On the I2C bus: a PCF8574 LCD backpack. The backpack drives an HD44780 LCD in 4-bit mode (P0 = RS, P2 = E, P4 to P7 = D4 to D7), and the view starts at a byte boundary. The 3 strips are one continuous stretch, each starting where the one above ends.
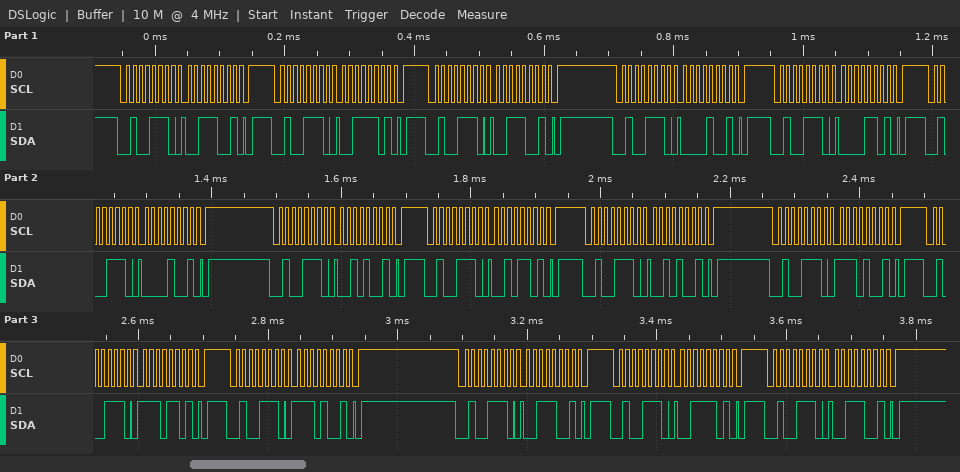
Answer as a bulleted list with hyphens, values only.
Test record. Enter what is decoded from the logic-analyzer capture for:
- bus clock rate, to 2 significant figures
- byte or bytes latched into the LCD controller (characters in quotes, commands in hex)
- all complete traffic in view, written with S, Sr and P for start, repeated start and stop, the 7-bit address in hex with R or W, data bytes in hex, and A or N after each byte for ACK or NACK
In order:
- 100 kHz
- '0' '.'
- S 27W A 39 A P S 27W A 3D A P S 27W A 39 A P S 27W A 09 A P S 27W A 0D A P S 27W A 09 A P S 27W A 29 A P S 27W A 2D A P S 27W A 29 A P S 27W A E9 A P S 27W A ED A P S 27W A E9 A P S 27W A 39 A P S 27W A 3D A P S 27W A 39 A P
